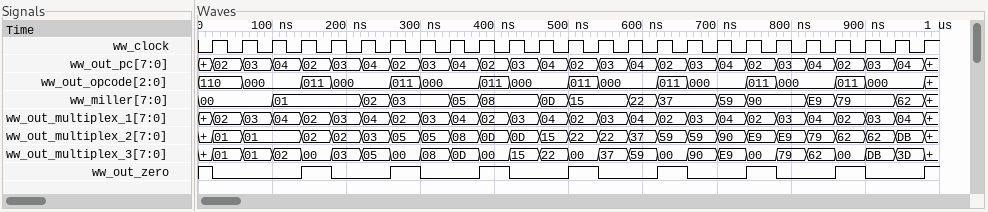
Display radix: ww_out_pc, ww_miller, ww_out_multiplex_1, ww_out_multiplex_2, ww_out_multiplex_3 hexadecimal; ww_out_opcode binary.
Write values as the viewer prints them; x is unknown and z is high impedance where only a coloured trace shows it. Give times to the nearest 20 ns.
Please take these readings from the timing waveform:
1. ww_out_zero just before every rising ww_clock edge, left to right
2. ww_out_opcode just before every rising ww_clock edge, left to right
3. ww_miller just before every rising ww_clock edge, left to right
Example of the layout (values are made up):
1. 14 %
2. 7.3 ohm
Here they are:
1. 1 0 0 0 1 0 0 1 0 0 1 0 0 1 0 0 1 0 0 1 0 0 1 0 0
2. 110, 110, 000, 000, 011, 000, 000, 011, 000, 000, 011, 000, 000, 011, 000, 000, 011, 000, 000, 011, 000, 000, 011, 000, 000
3. 00, 00, 00, 01, 01, 01, 02, 03, 03, 05, 08, 08, 0D, 15, 15, 22, 37, 37, 59, 90, 90, E9, 79, 79, 62
